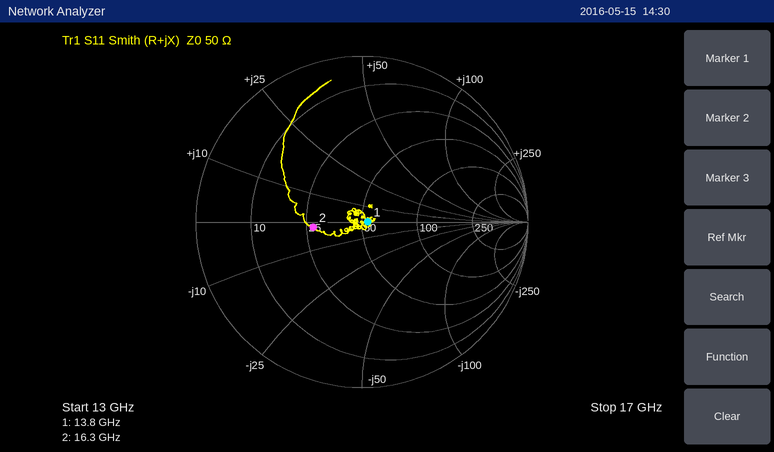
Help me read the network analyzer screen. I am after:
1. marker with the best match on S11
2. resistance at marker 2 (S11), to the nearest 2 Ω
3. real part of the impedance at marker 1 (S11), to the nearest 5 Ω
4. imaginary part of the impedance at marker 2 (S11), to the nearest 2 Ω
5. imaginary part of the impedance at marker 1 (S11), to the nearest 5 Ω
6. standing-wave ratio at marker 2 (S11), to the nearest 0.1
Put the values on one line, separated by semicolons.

marker 1; 28 Ω; 55 Ω; -2 Ω; 0 Ω; 1.8
